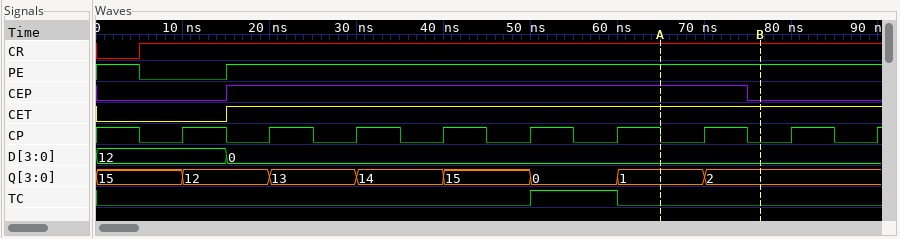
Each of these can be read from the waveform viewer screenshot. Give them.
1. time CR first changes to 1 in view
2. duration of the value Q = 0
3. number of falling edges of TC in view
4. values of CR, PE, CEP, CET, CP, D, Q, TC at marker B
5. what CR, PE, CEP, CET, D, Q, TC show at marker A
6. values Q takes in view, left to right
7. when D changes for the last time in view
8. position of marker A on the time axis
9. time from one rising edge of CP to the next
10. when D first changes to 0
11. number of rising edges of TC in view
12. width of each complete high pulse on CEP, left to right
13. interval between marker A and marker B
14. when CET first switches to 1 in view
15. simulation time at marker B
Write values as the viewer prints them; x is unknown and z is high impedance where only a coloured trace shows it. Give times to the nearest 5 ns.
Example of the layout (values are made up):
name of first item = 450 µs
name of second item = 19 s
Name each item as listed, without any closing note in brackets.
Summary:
time CR first changes to 1 in view = 5 ns
duration of the value Q = 0 = 10 ns
number of falling edges of TC in view = 1
values of CR, PE, CEP, CET, CP, D, Q, TC at marker B = CR=1, PE=1, CEP=0, CET=1, CP=0, D=0, Q=2, TC=0
what CR, PE, CEP, CET, D, Q, TC show at marker A = CR=1, PE=1, CEP=1, CET=1, D=0, Q=1, TC=0
values Q takes in view, left to right = 15, 12, 13, 14, 15, 0, 1, 2
when D changes for the last time in view = 15 ns
position of marker A on the time axis = 65 ns
time from one rising edge of CP to the next = 10 ns
when D first changes to 0 = 15 ns
number of rising edges of TC in view = 1
width of each complete high pulse on CEP, left to right = 60 ns
interval between marker A and marker B = 10 ns
when CET first switches to 1 in view = 15 ns
simulation time at marker B = 75 ns
